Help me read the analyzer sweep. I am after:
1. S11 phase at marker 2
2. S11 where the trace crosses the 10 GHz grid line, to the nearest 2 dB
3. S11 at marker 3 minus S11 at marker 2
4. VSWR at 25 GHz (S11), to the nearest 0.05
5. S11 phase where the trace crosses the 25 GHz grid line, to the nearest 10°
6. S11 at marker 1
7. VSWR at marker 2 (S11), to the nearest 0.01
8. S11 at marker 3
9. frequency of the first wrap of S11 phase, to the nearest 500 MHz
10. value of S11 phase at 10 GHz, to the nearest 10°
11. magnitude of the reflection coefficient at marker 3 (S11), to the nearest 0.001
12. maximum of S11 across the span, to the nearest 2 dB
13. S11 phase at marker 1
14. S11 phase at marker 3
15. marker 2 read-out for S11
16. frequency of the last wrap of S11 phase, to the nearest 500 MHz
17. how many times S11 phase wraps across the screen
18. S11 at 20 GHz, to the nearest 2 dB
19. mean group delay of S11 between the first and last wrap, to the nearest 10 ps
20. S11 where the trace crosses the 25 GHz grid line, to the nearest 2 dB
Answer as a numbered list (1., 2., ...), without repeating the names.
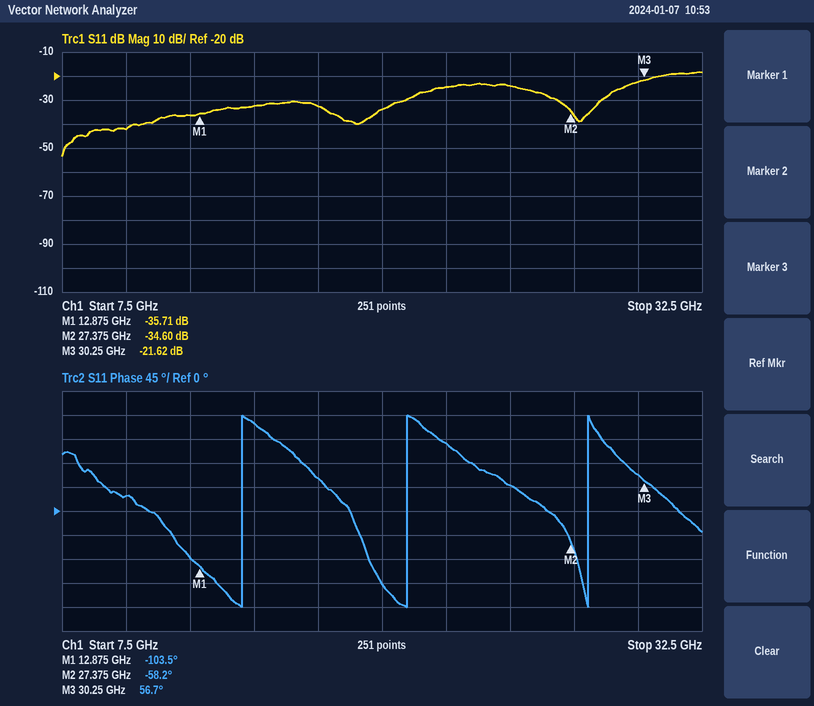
1. -58.2°
2. -42 dB
3. 12.98 dB
4. 1.15
5. 50°
6. -35.71 dB
7. 1.04
8. -21.62 dB
9. 14.5 GHz
10. 30°
11. 0.083
12. -18 dB
13. -103.5°
14. 56.7°
15. -34.60 dB
16. 28.0 GHz
17. 3
18. -34 dB
19. 150 ps
20. -24 dB
